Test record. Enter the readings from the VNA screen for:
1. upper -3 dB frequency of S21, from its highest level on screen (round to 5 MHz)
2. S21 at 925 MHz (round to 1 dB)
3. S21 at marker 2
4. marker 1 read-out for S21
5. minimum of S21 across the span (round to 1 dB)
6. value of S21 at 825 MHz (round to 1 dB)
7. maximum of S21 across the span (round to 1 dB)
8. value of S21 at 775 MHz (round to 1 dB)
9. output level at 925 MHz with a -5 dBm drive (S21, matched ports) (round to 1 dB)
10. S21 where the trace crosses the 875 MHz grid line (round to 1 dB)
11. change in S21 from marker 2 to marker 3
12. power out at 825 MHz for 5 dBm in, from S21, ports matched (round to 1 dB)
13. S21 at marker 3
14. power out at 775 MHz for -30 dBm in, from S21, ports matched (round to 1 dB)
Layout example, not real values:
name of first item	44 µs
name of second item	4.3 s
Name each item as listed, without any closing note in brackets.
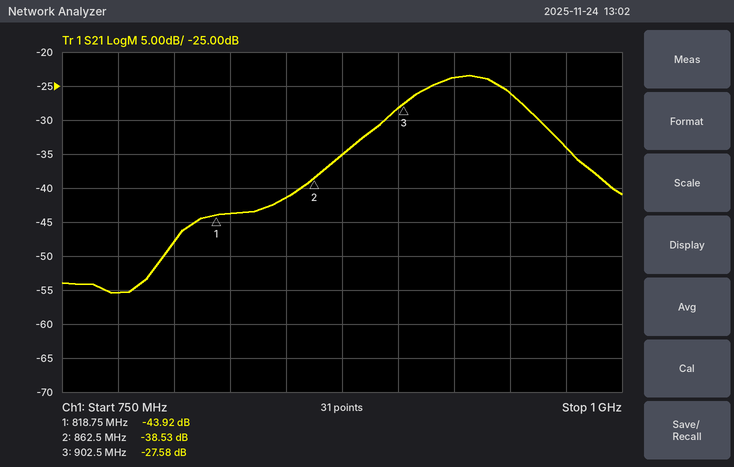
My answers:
upper -3 dB frequency of S21, from its highest level on screen	950 MHz
S21 at 925 MHz	-24 dB
S21 at marker 2	-38.53 dB
marker 1 read-out for S21	-43.92 dB
minimum of S21 across the span	-55 dB
value of S21 at 825 MHz	-44 dB
maximum of S21 across the span	-23 dB
value of S21 at 775 MHz	-55 dB
output level at 925 MHz with a -5 dBm drive (S21, matched ports)	-29 dBm
S21 where the trace crosses the 875 MHz grid line	-35 dB
change in S21 from marker 2 to marker 3	10.95 dB
power out at 825 MHz for 5 dBm in, from S21, ports matched	-39 dBm
S21 at marker 3	-27.58 dB
power out at 775 MHz for -30 dBm in, from S21, ports matched	-85 dBm
